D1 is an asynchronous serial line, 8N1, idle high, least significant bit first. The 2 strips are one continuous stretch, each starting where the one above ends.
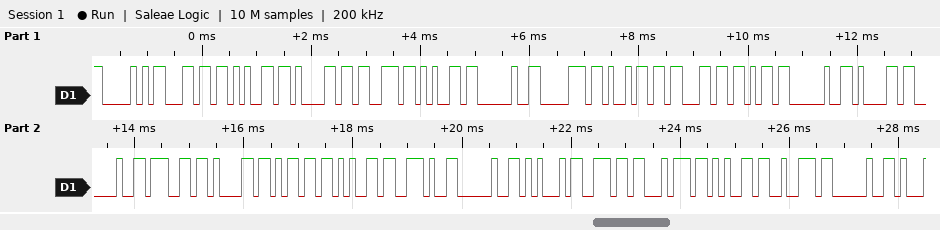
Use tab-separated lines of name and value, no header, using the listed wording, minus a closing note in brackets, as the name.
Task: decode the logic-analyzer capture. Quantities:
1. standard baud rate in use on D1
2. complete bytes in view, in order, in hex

standard baud rate in use on D1	9600 baud
complete bytes in view, in order, in hex	50 6C 65 61 73 65 20 70 69 63 6B 20 61 20 67 61 6D 65 2E 20 45 6E 74 65 72 20
